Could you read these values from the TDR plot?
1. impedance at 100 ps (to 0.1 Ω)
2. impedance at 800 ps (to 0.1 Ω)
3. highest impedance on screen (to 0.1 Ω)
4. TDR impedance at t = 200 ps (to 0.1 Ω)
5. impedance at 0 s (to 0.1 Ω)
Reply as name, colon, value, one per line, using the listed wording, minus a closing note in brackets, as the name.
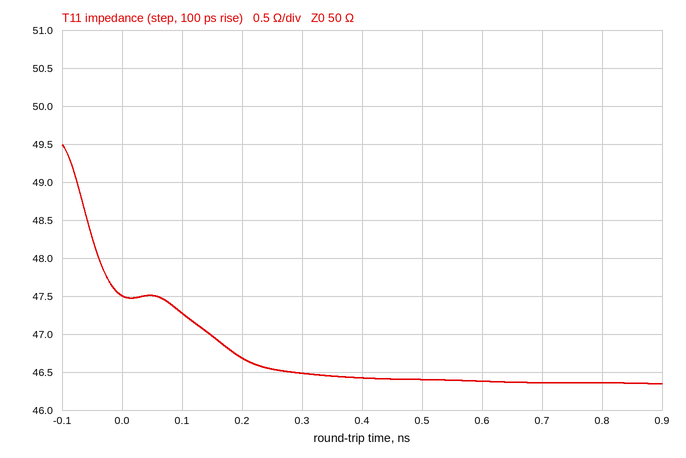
impedance at 100 ps: 47.3 Ω
impedance at 800 ps: 46.4 Ω
highest impedance on screen: 49.5 Ω
TDR impedance at t = 200 ps: 46.7 Ω
impedance at 0 s: 47.5 Ω
